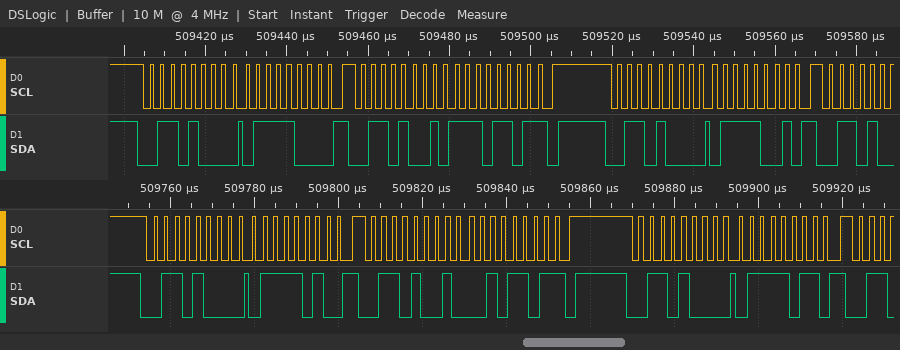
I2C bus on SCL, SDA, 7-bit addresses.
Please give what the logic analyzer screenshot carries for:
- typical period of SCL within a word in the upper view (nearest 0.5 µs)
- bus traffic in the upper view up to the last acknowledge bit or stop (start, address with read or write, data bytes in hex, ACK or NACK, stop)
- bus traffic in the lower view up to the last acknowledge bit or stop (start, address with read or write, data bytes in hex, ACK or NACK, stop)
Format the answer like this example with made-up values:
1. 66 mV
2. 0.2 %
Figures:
1. 2.5 µs
2. start, address 34 write ACK, 78 ACK, repeated start, address 34 read ACK, ED NACK, stop, start, address 34 write ACK, 79 ACK
3. start, address 34 write ACK, 7A ACK, repeated start, address 34 read ACK, 2D NACK, stop, start, address 34 write ACK, 7B ACK
